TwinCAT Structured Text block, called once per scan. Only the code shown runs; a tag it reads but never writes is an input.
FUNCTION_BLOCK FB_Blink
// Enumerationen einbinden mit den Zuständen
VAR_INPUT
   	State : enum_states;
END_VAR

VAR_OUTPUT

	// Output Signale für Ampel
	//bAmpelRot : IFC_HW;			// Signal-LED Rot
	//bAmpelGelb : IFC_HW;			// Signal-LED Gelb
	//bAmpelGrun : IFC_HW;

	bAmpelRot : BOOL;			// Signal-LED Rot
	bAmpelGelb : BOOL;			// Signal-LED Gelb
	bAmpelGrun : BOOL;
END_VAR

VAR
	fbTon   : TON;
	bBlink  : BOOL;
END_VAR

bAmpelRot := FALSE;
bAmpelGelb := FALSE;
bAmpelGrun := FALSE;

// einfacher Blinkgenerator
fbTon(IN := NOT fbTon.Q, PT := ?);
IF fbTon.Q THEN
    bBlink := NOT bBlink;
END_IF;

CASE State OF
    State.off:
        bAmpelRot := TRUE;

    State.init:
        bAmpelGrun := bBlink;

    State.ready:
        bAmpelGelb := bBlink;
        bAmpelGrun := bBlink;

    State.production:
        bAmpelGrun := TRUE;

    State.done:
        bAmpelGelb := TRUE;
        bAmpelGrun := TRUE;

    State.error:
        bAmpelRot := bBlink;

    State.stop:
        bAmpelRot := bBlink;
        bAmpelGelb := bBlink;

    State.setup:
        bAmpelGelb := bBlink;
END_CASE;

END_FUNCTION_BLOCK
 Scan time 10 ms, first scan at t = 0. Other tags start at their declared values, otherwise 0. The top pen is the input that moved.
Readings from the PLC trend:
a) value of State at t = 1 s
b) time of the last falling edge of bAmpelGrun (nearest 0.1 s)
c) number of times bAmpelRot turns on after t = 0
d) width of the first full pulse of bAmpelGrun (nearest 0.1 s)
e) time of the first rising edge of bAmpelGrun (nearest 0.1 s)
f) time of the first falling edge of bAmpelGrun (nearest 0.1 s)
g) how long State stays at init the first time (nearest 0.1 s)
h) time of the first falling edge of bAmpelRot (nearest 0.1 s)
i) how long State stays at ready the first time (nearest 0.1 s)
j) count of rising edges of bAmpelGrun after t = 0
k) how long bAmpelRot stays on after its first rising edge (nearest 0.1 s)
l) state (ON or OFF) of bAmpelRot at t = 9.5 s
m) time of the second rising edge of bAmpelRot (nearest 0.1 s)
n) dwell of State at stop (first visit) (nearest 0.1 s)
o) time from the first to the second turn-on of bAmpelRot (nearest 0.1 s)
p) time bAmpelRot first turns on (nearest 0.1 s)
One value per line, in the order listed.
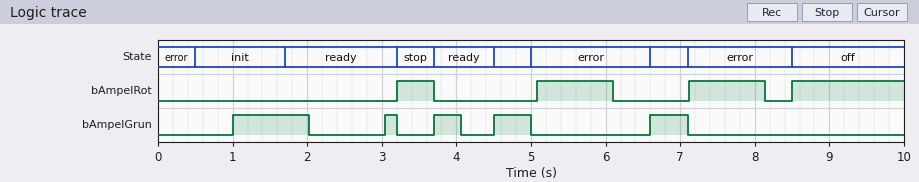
init
7.1 s
4
1.0 s
1.0 s
2.0 s
1.2 s
3.7 s
1.5 s
5
0.5 s
ON
5.1 s
0.5 s
1.9 s
3.2 s
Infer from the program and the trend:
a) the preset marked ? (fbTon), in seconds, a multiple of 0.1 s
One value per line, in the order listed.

1.0 s
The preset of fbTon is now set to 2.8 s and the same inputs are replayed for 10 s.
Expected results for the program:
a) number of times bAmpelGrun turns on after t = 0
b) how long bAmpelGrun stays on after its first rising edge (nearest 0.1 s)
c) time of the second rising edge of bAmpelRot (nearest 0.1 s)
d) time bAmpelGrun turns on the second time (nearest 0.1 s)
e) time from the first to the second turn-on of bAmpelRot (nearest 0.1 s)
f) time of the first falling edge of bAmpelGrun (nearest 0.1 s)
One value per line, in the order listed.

3
0.4 s
5.0 s
3.7 s
1.8 s
3.2 s
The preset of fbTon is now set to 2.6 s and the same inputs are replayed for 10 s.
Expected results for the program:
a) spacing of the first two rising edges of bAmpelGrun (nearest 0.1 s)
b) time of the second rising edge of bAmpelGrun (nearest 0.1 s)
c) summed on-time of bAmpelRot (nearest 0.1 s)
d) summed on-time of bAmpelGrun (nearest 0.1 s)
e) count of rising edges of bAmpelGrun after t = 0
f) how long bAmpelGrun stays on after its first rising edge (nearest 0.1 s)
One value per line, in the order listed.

1.1 s
3.7 s
2.9 s
2.4 s
3
0.6 s
